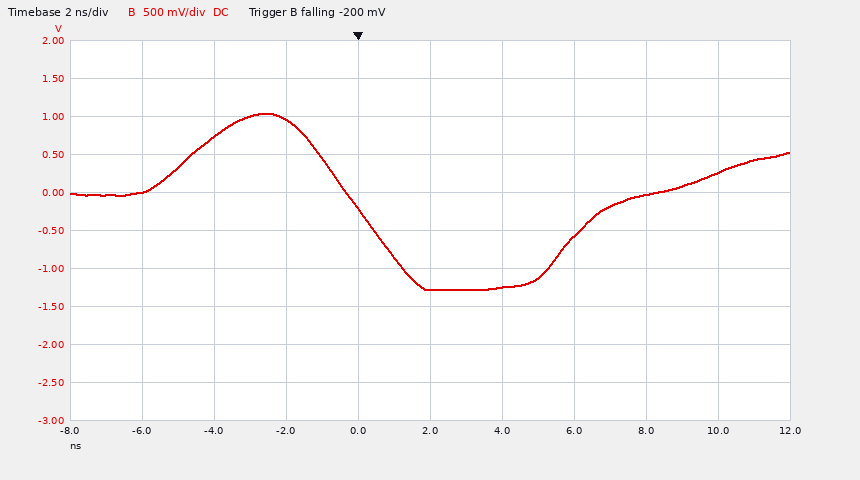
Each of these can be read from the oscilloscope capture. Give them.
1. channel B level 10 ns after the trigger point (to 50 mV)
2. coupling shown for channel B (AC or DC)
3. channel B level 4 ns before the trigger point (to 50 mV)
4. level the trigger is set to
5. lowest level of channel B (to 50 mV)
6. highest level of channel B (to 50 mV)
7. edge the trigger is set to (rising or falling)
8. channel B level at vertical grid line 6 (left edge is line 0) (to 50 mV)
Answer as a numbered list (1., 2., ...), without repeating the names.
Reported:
1. 250 mV
2. DC
3. 750 mV
4. -200 mV
5. -1.30 V
6. 1.05 V
7. falling
8. -1.25 V
